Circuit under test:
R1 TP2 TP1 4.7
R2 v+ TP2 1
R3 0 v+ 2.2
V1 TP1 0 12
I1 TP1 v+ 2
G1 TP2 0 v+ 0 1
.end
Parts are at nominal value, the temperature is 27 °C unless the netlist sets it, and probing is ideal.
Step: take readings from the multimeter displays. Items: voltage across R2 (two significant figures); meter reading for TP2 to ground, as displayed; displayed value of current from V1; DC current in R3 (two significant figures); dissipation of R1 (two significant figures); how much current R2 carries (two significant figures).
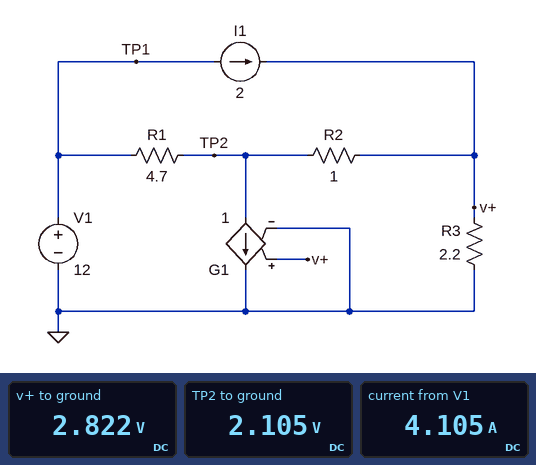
720 mV
2.105 V
4.105 A
1.3 A
21 W
720 mA
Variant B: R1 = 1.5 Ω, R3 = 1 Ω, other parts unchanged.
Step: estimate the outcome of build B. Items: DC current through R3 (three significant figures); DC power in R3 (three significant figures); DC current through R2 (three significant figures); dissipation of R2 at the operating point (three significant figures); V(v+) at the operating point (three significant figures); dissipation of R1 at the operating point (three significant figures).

3.40 A
11.6 W
1.40 A
1.96 W
3.40 V
34.6 W
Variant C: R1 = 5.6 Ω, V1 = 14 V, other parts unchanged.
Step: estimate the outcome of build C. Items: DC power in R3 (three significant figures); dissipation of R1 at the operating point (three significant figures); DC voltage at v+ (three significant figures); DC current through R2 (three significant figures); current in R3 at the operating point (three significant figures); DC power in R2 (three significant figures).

3.65 W
25.2 W
2.83 V
712 mA
1.29 A
507 mW
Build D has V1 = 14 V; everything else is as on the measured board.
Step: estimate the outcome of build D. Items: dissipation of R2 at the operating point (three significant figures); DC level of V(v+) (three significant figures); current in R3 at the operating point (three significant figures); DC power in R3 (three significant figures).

369 mW
3.06 V
1.39 A
4.27 W
